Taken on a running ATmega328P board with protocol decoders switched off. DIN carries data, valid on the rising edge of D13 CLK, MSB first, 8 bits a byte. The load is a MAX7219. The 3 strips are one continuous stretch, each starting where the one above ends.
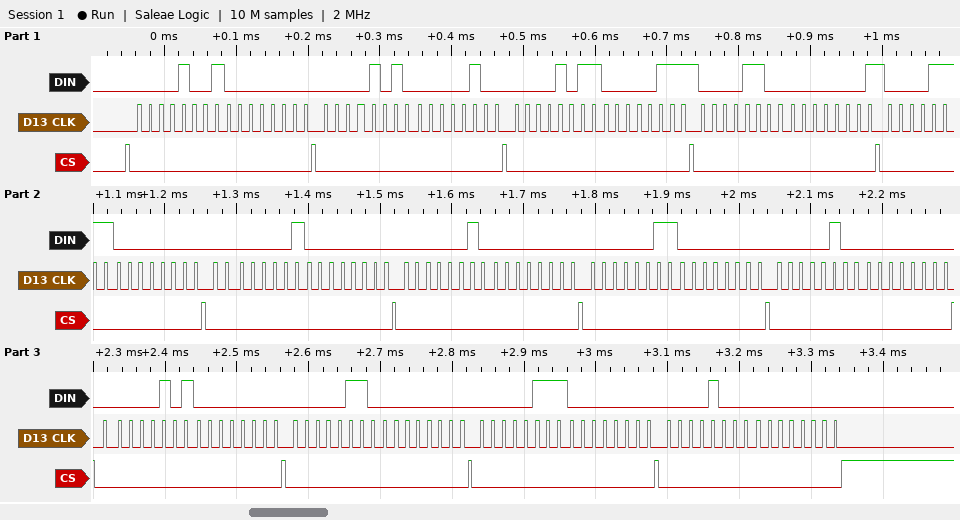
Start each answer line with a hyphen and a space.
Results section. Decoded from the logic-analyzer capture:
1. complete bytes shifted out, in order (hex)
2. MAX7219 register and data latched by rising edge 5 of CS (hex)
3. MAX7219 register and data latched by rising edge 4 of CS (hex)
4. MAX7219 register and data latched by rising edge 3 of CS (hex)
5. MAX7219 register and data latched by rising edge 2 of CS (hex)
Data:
- 09 00 0A 04 0B 07 0C 01 0F 00 01 00 02 00 03 00 04 00 05 00 06 00 07 00 08 00
- register 0xC, data 0x01
- register 0xB, data 0x07
- register 0xA, data 0x04
- register 0x9, data 0x00
